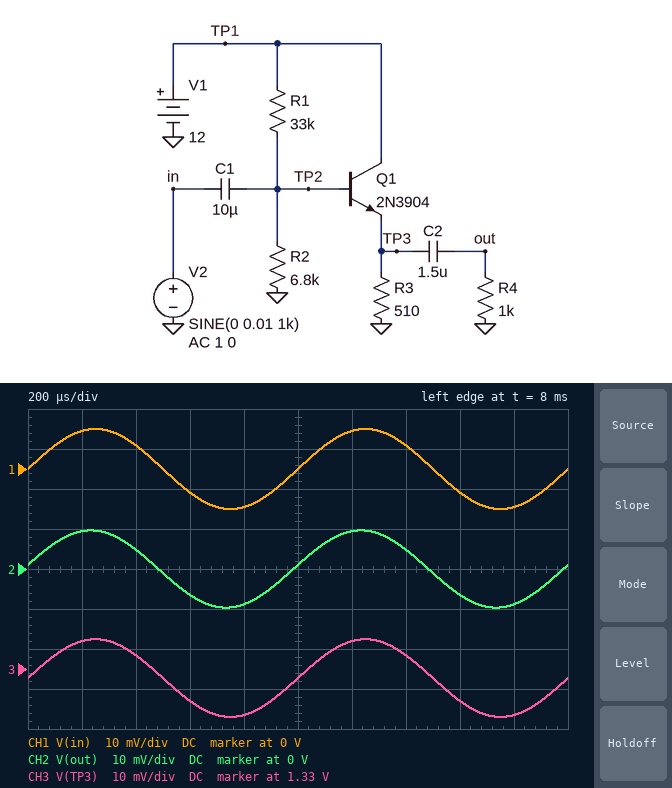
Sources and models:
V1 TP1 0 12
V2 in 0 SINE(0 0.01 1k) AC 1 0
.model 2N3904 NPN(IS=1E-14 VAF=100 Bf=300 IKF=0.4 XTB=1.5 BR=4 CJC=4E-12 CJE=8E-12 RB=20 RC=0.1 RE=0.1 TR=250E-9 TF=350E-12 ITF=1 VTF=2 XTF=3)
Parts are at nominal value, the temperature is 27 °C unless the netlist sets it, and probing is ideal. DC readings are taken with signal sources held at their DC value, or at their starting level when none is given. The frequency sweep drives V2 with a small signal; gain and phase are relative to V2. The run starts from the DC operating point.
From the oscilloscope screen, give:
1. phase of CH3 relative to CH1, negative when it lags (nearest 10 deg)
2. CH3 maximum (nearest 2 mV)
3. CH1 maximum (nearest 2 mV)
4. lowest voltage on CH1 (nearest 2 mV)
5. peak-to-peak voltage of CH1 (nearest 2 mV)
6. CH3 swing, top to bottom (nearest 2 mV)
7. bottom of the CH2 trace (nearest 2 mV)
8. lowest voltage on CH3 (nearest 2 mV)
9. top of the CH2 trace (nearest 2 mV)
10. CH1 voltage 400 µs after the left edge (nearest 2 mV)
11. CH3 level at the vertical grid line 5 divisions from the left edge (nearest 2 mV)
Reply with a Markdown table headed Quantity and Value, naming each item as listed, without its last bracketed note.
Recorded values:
| Quantity | Value |
|---|---|
| phase of CH3 relative to CH1, negative when it lags | 0 deg |
| CH3 maximum | 1.338 V |
| CH1 maximum | 10 mV |
| lowest voltage on CH1 | -10 mV |
| peak-to-peak voltage of CH1 | 20 mV |
| CH3 swing, top to bottom | 20 mV |
| bottom of the CH2 trace | -10 mV |
| lowest voltage on CH3 | 1.318 V |
| top of the CH2 trace | 10 mV |
| CH1 voltage 400 µs after the left edge | 6 mV |
| CH3 level at the vertical grid line 5 divisions from the left edge | 1.328 V |
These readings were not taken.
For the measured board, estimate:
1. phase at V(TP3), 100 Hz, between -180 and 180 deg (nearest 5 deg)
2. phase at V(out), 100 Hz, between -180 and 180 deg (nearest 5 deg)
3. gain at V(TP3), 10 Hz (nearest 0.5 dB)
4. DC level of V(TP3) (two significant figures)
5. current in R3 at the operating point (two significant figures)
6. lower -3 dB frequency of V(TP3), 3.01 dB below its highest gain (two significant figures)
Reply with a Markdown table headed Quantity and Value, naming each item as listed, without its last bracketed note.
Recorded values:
| Quantity | Value |
|---|---|
| phase at V(TP3), 100 Hz, between -180 and 180 deg | 0 deg |
| phase at V(out), 100 Hz, between -180 and 180 deg | 50 deg |
| gain at V(TP3), 10 Hz | -0.5 dB |
| DC level of V(TP3) | 1.3 V |
| current in R3 at the operating point | 2.6 mA |
| lower -3 dB frequency of V(TP3), 3.01 dB below its highest gain | 2.9 Hz |
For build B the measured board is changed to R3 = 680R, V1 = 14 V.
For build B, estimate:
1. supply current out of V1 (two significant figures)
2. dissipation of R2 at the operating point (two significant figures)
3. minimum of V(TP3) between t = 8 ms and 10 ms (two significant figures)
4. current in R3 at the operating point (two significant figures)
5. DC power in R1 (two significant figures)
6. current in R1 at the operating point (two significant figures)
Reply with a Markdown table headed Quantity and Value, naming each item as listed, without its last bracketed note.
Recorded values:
| Quantity | Value |
|---|---|
| supply current out of V1 | 2.8 mA |
| dissipation of R2 at the operating point | 810 µW |
| minimum of V(TP3) between t = 8 ms and 10 ms | 1.7 V |
| current in R3 at the operating point | 2.5 mA |
| DC power in R1 | 4.1 mW |
| current in R1 at the operating point | 350 µA |
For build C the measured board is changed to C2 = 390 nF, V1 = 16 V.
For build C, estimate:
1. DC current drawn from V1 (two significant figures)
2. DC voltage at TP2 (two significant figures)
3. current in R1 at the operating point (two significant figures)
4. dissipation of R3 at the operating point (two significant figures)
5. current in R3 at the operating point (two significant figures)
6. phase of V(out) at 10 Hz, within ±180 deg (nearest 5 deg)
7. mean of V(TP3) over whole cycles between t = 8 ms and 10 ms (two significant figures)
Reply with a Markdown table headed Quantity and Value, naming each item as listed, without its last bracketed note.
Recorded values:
| Quantity | Value |
|---|---|
| DC current drawn from V1 | 4.3 mA |
| DC voltage at TP2 | 2.7 V |
| current in R1 at the operating point | 400 µA |
| dissipation of R3 at the operating point | 7.7 mW |
| current in R3 at the operating point | 3.9 mA |
| phase of V(out) at 10 Hz, within ±180 deg | 105 deg |
| mean of V(TP3) over whole cycles between t = 8 ms and 10 ms | 2.0 V |
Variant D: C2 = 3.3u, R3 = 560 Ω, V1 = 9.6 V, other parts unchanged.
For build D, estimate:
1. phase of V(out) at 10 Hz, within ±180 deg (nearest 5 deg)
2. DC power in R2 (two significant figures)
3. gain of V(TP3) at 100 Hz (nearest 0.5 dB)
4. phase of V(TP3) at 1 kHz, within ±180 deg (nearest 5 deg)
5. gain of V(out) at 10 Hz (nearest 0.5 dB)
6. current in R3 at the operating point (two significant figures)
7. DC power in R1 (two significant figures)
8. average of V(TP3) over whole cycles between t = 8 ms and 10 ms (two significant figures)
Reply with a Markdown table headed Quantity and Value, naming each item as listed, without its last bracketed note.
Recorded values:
| Quantity | Value |
|---|---|
| phase of V(out) at 10 Hz, within ±180 deg | 95 deg |
| DC power in R2 | 380 µW |
| gain of V(TP3) at 100 Hz | -0.5 dB |
| phase of V(TP3) at 1 kHz, within ±180 deg | 0 deg |
| gain of V(out) at 10 Hz | -14.5 dB |
| current in R3 at the operating point | 1.7 mA |
| DC power in R1 | 1.9 mW |
| average of V(TP3) over whole cycles between t = 8 ms and 10 ms | 940 mV |
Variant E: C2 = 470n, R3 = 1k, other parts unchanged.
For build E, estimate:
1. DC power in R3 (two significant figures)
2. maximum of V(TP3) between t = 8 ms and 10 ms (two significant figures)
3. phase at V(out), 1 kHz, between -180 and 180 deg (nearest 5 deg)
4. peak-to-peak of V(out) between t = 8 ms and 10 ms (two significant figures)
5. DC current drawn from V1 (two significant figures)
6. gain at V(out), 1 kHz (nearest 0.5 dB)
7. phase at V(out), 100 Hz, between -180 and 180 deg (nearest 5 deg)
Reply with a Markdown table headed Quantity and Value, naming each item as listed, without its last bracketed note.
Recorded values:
| Quantity | Value |
|---|---|
| DC power in R3 | 1.9 mW |
| maximum of V(TP3) between t = 8 ms and 10 ms | 1.4 V |
| phase at V(out), 1 kHz, between -180 and 180 deg | 20 deg |
| peak-to-peak of V(out) between t = 8 ms and 10 ms | 18 mV |
| DC current drawn from V1 | 1.7 mA |
| gain at V(out), 1 kHz | -1.0 dB |
| phase at V(out), 100 Hz, between -180 and 180 deg | 75 deg |
